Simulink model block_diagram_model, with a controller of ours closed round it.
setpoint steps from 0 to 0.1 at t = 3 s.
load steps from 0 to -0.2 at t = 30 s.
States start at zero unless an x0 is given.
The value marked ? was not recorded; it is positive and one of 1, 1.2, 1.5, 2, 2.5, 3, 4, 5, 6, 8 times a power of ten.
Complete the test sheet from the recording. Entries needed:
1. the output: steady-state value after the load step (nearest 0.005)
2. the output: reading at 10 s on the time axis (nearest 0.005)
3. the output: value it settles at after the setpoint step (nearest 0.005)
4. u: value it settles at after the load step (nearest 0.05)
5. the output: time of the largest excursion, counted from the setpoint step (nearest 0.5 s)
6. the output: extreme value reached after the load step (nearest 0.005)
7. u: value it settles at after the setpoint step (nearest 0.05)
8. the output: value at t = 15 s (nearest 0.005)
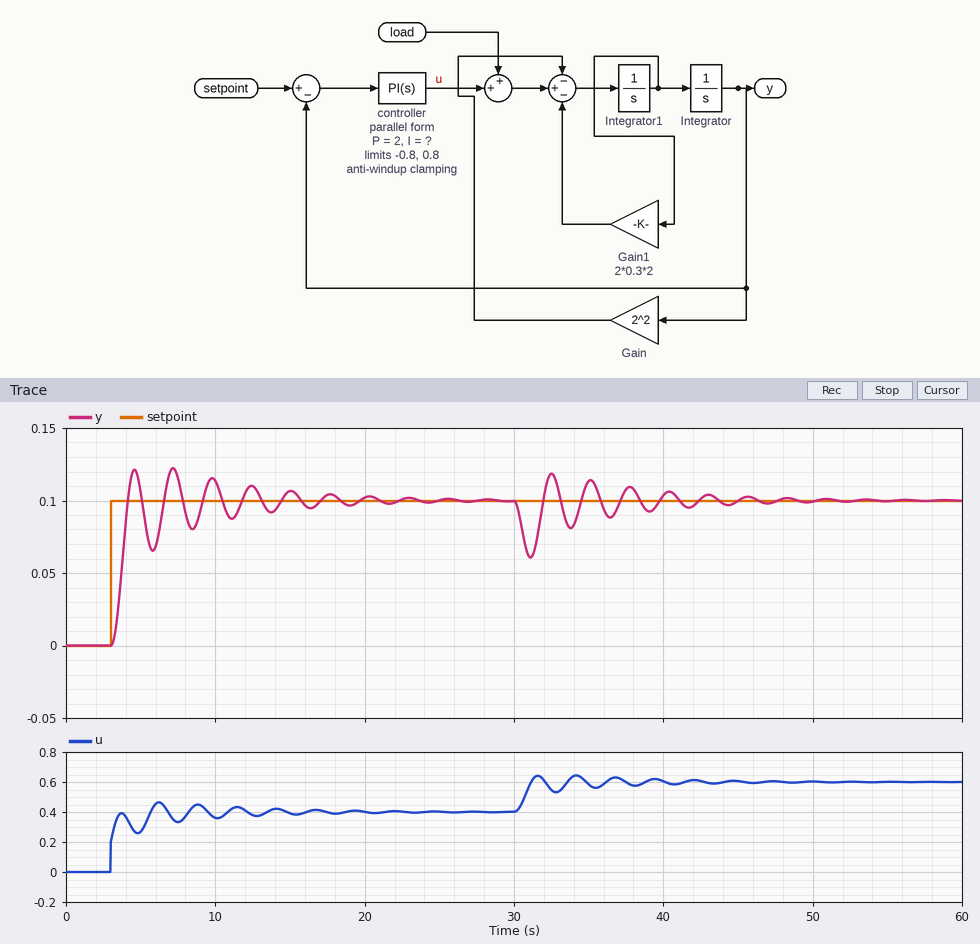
0.100
0.115
0.100
0.60
4.0 s
0.060
0.40
0.105
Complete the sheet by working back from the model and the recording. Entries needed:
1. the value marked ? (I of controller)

5
